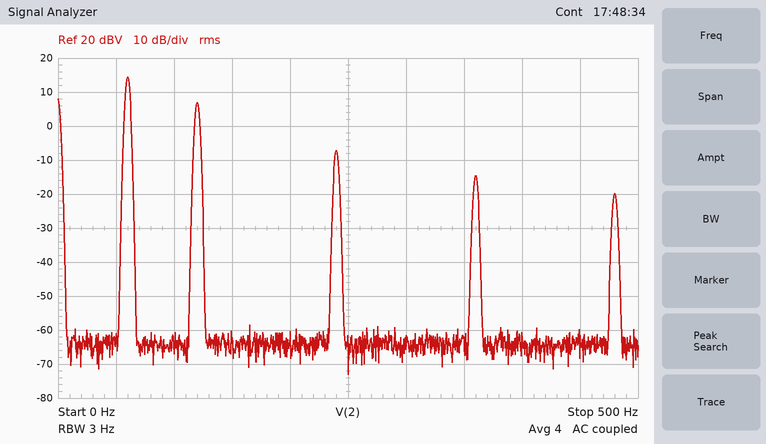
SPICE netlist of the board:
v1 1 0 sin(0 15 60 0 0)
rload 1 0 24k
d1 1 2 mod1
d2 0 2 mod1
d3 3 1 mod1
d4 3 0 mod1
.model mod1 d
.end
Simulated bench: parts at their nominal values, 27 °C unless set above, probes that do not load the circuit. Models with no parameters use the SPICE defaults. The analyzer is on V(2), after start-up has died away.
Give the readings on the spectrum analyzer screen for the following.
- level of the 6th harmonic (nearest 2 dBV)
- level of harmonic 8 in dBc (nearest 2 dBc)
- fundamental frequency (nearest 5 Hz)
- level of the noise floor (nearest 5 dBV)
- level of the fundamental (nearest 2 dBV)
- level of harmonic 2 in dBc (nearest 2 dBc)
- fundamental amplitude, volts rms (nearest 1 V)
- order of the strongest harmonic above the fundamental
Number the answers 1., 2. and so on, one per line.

1. -14 dBV
2. -34 dBc
3. 60 Hz
4. -65 dBV
5. 14 dBV
6. -8 dBc
7. 5 V
8. 2
